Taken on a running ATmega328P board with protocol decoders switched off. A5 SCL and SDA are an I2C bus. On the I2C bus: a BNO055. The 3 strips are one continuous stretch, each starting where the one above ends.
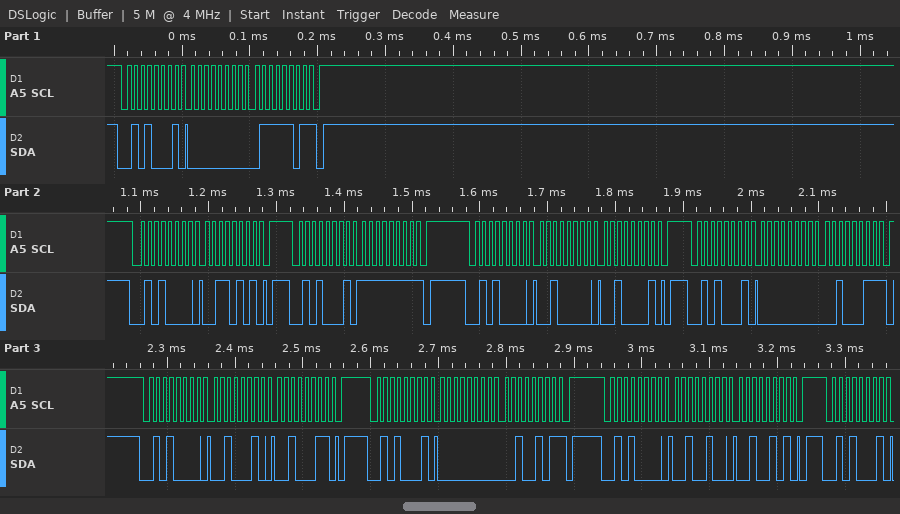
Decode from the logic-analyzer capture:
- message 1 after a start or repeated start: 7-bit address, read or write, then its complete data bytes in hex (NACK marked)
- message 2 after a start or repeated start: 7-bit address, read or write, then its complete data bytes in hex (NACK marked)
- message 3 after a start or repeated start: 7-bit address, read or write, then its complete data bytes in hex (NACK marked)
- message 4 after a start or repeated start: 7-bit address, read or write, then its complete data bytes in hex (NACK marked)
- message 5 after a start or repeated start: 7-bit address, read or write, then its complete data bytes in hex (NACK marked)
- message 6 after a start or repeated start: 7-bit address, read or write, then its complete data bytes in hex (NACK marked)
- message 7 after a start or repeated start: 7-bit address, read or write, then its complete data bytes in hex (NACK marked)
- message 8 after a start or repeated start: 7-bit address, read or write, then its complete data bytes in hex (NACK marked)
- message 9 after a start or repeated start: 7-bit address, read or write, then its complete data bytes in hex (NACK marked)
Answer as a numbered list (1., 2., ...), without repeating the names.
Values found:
1. 0x28 read: 00 7D NACK
2. 0x28 write: 35
3. 0x28 read: FF NACK
4. 0x28 write: 20 21
5. 0x28 read: 00 23 NACK
6. 0x28 write: 22 23
7. 0x28 read: 00 25 NACK
8. 0x28 write: 24 25
9. 0x28 read
